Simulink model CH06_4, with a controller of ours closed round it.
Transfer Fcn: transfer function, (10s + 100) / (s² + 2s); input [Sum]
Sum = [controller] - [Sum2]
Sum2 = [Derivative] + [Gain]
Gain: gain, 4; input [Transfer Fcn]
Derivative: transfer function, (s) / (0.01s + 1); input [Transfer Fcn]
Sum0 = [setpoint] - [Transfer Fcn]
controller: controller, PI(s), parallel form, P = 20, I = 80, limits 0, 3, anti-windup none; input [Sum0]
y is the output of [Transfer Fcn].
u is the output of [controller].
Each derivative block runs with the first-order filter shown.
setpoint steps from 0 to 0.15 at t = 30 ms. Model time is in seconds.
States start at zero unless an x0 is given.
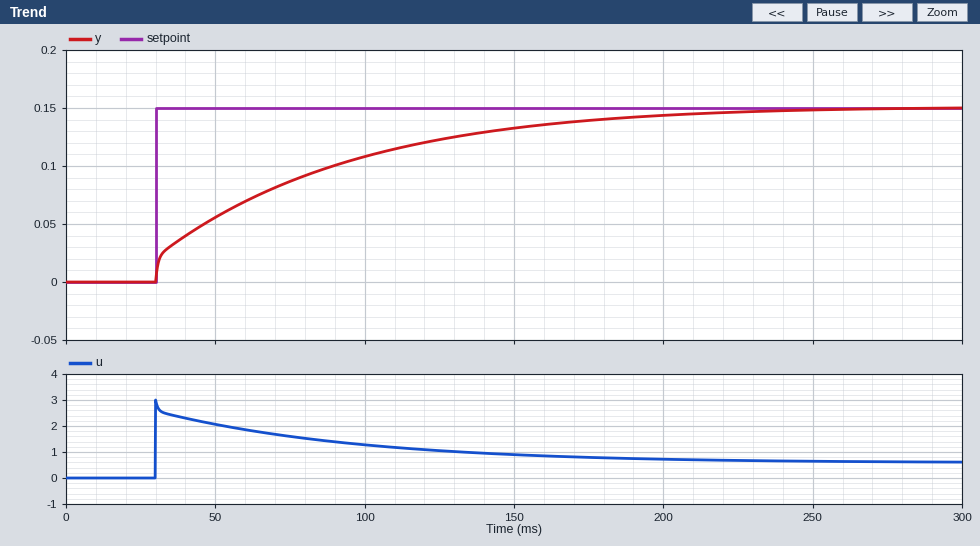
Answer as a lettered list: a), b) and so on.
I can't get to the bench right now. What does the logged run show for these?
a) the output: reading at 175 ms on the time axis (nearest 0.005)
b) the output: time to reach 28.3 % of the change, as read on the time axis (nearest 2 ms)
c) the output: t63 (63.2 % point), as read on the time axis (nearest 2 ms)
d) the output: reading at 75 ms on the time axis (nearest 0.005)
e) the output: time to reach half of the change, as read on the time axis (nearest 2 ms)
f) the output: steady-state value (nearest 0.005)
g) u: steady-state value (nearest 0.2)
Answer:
a) 0.140
b) 42 ms
c) 84 ms
d) 0.085
e) 64 ms
f) 0.150
g) 0.6
